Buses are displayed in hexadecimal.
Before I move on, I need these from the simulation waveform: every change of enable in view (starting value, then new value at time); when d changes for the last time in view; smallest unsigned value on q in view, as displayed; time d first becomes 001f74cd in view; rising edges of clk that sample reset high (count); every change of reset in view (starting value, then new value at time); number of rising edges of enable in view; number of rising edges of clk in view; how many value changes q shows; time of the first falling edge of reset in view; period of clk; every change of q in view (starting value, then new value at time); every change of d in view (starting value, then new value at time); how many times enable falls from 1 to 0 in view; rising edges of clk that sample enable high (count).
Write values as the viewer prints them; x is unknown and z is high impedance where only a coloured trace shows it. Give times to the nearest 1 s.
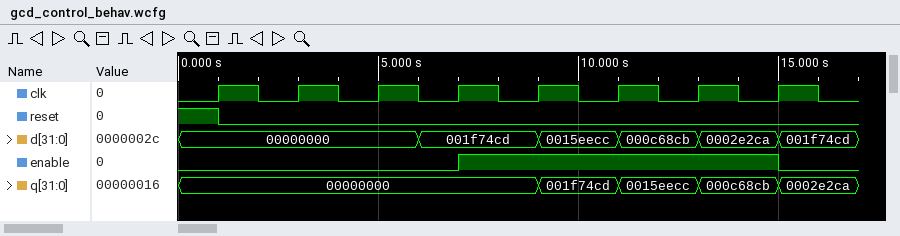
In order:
0, 1 at 7 s, 0 at 15 s
15 s
00000000
6 s
1
1, 0 at 1 s
1
8
4
1 s
2 s
00000000, 001f74cd at 9 s, 0015eecc at 11 s, 000c68cb at 13 s, 0002e2ca at 15 s
00000000, 001f74cd at 6 s, 0015eecc at 9 s, 000c68cb at 11 s, 0002e2ca at 13 s, 001f74cd at 15 s
1
4
